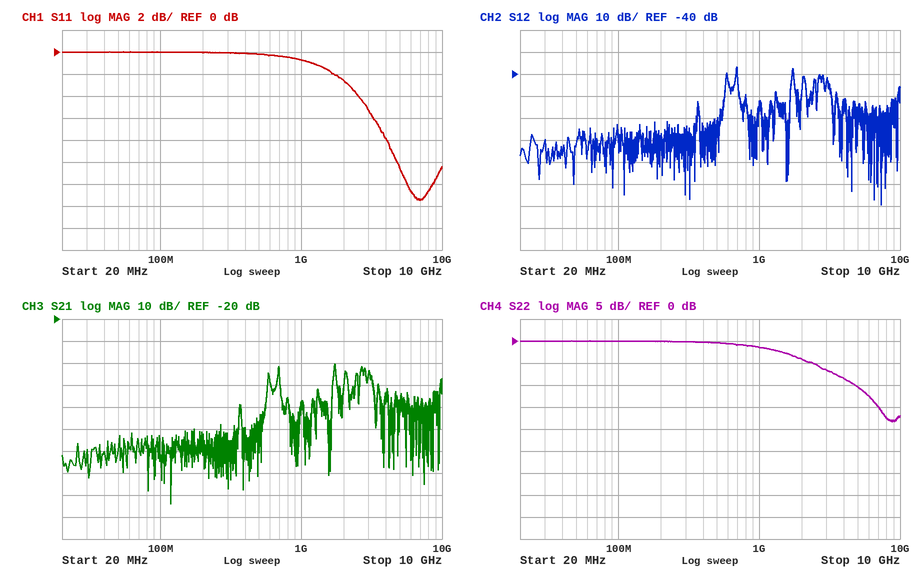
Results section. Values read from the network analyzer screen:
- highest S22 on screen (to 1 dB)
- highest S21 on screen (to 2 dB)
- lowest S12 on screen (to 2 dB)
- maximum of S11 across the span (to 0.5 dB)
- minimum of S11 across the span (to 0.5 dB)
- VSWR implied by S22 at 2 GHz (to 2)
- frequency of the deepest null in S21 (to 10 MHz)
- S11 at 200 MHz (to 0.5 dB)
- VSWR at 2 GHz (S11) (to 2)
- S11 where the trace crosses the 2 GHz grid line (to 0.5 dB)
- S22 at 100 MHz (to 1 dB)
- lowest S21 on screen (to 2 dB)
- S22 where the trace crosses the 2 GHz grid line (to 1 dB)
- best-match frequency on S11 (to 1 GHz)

0 dB
-40 dB
-100 dB
0.0 dB
-13.5 dB
4
120 MHz
0.0 dB
6
-2.5 dB
0 dB
-104 dB
-4 dB
7 GHz
